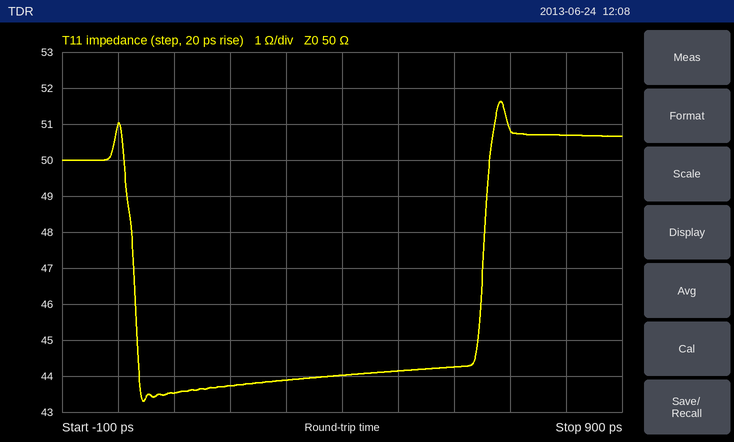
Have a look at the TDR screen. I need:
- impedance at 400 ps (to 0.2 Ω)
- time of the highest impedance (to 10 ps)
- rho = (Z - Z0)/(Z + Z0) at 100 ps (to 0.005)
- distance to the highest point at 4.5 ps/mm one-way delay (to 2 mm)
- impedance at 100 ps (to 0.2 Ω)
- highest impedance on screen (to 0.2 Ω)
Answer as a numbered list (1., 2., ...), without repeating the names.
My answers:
1. 44.0 Ω
2. 680 ps
3. -0.070
4. 76 mm
5. 43.6 Ω
6. 51.6 Ω
